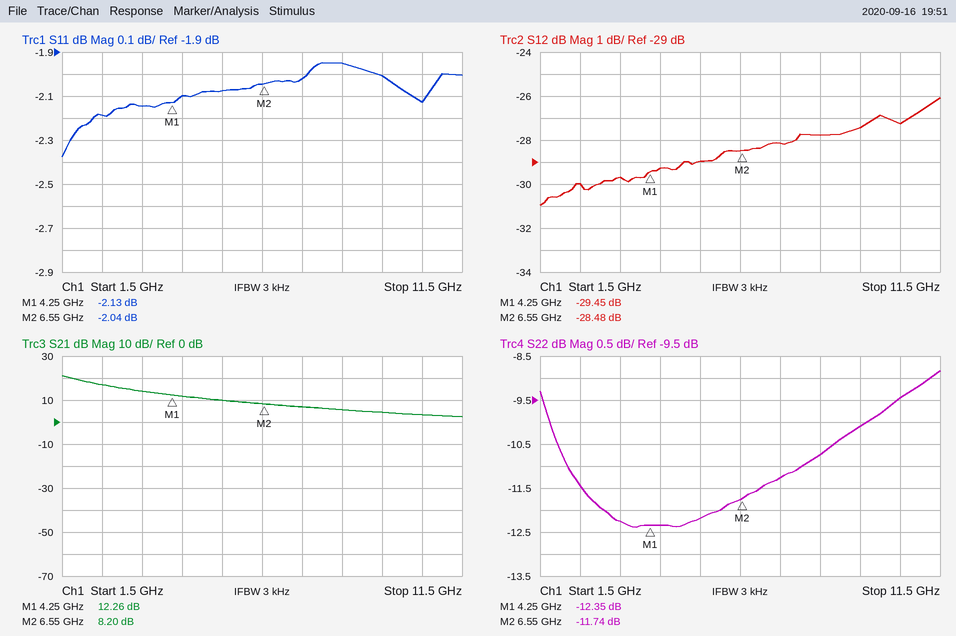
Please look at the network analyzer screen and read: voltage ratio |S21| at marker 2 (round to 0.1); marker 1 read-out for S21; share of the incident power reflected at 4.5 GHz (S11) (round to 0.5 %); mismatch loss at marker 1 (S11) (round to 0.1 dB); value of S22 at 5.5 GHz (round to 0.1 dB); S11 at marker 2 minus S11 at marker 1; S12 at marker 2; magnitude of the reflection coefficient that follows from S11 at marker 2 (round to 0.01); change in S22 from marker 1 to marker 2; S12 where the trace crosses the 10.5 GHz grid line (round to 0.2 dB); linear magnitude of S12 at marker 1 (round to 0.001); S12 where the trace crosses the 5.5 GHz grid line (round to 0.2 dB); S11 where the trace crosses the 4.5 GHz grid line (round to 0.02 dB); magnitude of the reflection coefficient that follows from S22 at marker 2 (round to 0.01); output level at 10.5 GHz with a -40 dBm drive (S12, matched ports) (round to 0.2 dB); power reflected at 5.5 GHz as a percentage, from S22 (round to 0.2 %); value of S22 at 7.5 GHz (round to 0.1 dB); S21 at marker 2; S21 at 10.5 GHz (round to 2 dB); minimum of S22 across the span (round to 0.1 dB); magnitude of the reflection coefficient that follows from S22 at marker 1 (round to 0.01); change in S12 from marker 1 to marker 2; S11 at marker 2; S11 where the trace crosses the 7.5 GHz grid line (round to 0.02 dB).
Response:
2.6
12.26 dB
61.5 %
4.1 dB
-12.2 dB
0.09 dB
-28.48 dB
0.79
0.61 dB
-27.2 dB
0.034
-29.0 dB
-2.10 dB
0.26
-67.2 dBm
6.0 %
-11.3 dB
8.20 dB
4 dB
-12.4 dB
0.24
0.97 dB
-2.04 dB
-2.02 dB
